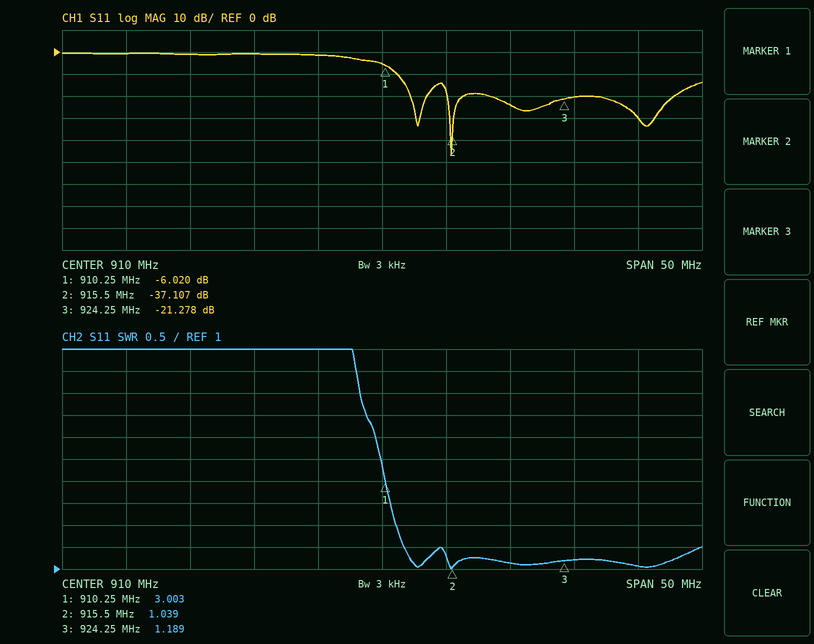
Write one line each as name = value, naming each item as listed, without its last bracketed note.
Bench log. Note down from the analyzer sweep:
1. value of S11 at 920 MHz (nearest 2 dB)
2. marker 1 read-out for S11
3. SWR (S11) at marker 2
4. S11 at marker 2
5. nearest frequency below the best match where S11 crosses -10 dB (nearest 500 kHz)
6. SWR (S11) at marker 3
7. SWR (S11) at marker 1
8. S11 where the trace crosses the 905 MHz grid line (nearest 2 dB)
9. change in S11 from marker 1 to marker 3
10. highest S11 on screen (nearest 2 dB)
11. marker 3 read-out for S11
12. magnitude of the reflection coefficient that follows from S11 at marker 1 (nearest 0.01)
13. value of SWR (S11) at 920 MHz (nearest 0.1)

value of S11 at 920 MHz = -24 dB
marker 1 read-out for S11 = -6.020 dB
SWR (S11) at marker 2 = 1.039
S11 at marker 2 = -37.107 dB
nearest frequency below the best match where S11 crosses -10 dB = 911.0 MHz
SWR (S11) at marker 3 = 1.189
SWR (S11) at marker 1 = 3.003
S11 where the trace crosses the 905 MHz grid line = -2 dB
change in S11 from marker 1 to marker 3 = -15.258 dB
highest S11 on screen = 0 dB
marker 3 read-out for S11 = -21.278 dB
magnitude of the reflection coefficient that follows from S11 at marker 1 = 0.50
value of SWR (S11) at 920 MHz = 1.1
